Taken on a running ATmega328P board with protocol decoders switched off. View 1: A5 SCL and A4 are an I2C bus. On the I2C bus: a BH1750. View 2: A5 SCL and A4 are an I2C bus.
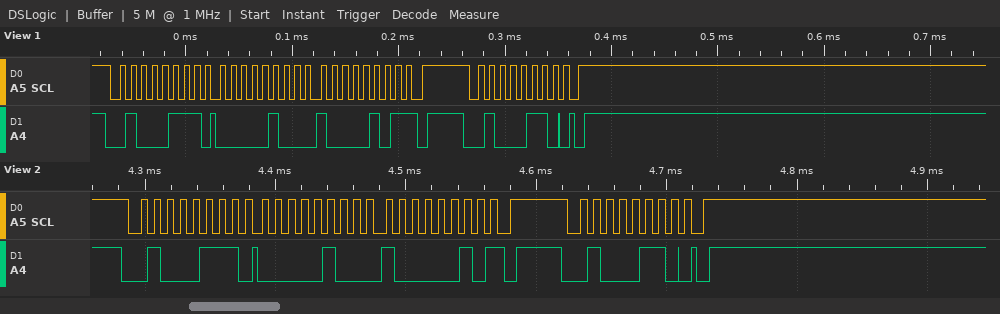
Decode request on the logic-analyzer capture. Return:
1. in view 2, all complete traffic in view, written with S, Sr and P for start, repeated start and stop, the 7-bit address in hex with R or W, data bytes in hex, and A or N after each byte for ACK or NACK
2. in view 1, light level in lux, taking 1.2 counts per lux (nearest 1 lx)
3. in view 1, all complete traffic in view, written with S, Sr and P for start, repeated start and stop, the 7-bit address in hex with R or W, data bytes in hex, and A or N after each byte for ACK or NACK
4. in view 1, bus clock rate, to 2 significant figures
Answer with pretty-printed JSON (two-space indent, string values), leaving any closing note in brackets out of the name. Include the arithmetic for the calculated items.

{
  "in view 2, all complete traffic in view, written with S, Sr and P for start, repeated start and stop, the 7-bit address in hex with R or W, data bytes in hex, and A or N after each byte for ACK or NACK": "S 23R A 04 A 82 N P S 23W A P",
  "in view 1, light level in lux, taking 1.2 counts per lux": "1157 / 1.2 = 964 lx",
  "in view 1, all complete traffic in view, written with S, Sr and P for start, repeated start and stop, the 7-bit address in hex with R or W, data bytes in hex, and A or N after each byte for ACK or NACK": "S 23R A 04 A 85 N P S 23W A P",
  "in view 1, bus clock rate, to 2 significant figures": "100 kHz"
}
